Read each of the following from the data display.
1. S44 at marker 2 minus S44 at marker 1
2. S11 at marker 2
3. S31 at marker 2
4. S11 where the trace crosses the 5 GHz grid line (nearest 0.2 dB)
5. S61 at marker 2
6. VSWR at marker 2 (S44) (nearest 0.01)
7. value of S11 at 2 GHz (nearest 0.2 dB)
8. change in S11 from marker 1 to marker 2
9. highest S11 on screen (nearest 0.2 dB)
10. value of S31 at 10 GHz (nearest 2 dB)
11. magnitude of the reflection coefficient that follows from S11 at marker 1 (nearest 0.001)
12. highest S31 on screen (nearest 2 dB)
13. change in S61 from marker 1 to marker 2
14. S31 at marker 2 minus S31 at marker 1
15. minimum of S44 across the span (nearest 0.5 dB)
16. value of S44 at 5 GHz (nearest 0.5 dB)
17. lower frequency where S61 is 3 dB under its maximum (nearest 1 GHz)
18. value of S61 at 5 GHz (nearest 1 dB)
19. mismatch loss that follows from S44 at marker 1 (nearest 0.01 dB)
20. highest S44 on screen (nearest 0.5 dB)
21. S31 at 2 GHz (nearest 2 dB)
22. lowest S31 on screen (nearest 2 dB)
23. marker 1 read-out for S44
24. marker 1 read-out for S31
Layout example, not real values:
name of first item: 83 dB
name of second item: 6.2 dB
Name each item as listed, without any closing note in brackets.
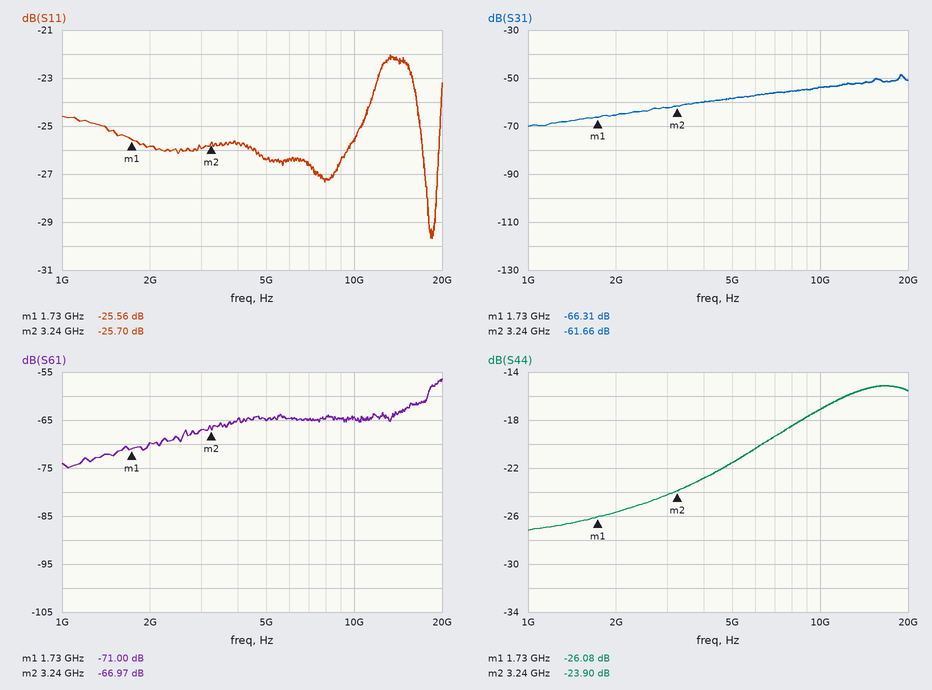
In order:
S44 at marker 2 minus S44 at marker 1: 2.18 dB
S11 at marker 2: -25.70 dB
S31 at marker 2: -61.66 dB
S11 where the trace crosses the 5 GHz grid line: -26.4 dB
S61 at marker 2: -66.97 dB
VSWR at marker 2 (S44): 1.14
value of S11 at 2 GHz: -25.8 dB
change in S11 from marker 1 to marker 2: -0.14 dB
highest S11 on screen: -22.0 dB
value of S31 at 10 GHz: -54 dB
magnitude of the reflection coefficient that follows from S11 at marker 1: 0.053
highest S31 on screen: -48 dB
change in S61 from marker 1 to marker 2: 4.03 dB
S31 at marker 2 minus S31 at marker 1: 4.65 dB
minimum of S44 across the span: -27.0 dB
value of S44 at 5 GHz: -21.5 dB
lower frequency where S61 is 3 dB under its maximum: 18 GHz
value of S61 at 5 GHz: -65 dB
mismatch loss that follows from S44 at marker 1: 0.01 dB
highest S44 on screen: -15.0 dB
S31 at 2 GHz: -66 dB
lowest S31 on screen: -70 dB
marker 1 read-out for S44: -26.08 dB
marker 1 read-out for S31: -66.31 dB
